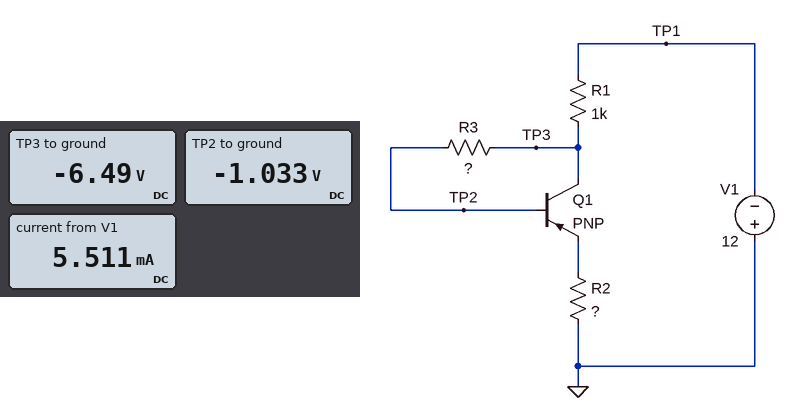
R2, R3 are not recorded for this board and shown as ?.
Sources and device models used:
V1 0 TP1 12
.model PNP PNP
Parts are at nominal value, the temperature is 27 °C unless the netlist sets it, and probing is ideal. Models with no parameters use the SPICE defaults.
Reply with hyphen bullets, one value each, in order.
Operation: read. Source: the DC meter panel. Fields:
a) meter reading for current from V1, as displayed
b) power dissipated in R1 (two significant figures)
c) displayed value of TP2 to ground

- 5.511 mA
- 30 mW
- -1.033 V
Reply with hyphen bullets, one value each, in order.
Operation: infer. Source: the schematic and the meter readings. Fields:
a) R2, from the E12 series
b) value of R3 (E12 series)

- 39 Ω
- 100 kΩ
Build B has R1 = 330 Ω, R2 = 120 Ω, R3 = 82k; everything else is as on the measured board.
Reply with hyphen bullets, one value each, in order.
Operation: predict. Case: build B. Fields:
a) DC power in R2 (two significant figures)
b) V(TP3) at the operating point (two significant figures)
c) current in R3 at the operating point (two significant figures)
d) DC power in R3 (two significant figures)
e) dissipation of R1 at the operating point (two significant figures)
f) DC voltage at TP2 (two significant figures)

- 9.4 mW
- -9.1 V
- 88 µA
- 630 µW
- 26 mW
- -1.9 V
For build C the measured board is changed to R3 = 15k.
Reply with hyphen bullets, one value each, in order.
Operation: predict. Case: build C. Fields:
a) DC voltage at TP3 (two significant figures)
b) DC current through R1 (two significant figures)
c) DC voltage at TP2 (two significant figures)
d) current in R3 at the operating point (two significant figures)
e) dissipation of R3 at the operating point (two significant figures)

- -2.6 V
- 9.4 mA
- -1.2 V
- 93 µA
- 130 µW
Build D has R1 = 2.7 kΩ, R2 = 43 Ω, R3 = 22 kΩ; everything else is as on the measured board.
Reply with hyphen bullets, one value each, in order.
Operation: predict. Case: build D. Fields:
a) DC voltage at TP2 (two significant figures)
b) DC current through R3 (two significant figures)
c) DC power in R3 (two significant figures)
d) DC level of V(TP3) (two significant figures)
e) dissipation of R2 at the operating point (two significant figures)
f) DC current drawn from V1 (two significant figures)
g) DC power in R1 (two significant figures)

- -970 mV
- 37 µA
- 31 µW
- -1.8 V
- 610 µW
- 3.8 mA
- 39 mW
